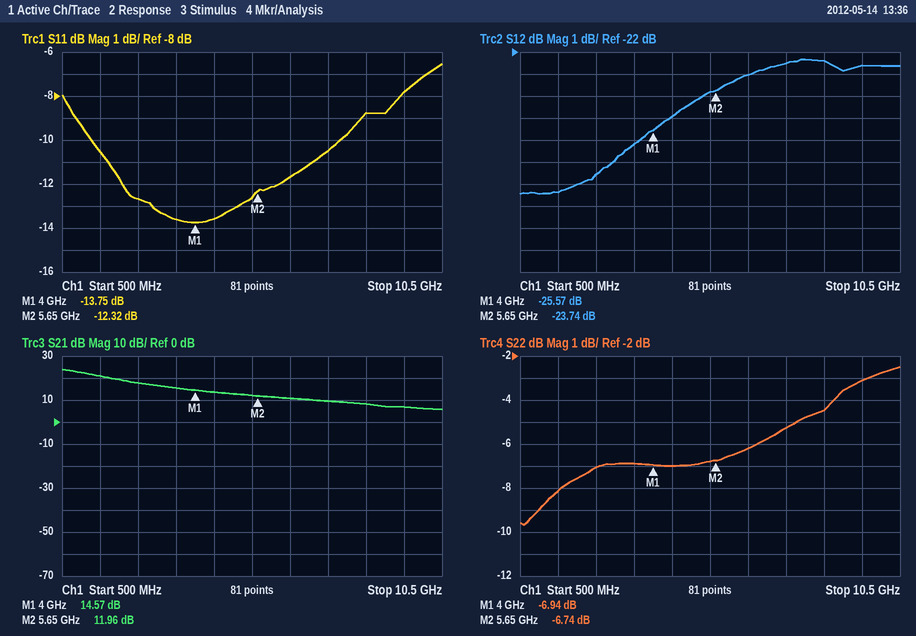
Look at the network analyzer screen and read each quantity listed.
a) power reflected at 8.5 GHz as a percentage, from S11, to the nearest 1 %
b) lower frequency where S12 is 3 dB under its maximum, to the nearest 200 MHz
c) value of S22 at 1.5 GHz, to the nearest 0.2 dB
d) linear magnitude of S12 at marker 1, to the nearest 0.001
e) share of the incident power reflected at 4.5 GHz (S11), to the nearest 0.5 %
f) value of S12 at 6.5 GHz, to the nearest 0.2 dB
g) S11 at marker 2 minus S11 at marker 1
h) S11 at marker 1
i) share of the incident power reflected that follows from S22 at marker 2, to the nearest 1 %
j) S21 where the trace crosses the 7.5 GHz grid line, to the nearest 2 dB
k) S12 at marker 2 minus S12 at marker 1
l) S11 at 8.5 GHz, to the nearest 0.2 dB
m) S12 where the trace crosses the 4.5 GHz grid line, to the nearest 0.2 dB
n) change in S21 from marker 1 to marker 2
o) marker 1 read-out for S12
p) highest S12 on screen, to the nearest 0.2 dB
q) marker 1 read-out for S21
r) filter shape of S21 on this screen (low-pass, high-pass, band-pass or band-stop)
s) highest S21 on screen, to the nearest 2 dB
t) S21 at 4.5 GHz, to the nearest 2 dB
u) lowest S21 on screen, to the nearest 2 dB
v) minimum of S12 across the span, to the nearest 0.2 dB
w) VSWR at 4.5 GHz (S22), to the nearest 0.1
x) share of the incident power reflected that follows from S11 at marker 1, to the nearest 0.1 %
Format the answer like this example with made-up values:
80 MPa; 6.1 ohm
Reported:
13 %; 4.2 GHz; -8.2 dB; 0.053; 4.5 %; -23.0 dB; 1.43 dB; -13.75 dB; 21 %; 10 dB; 1.83 dB; -8.8 dB; -25.0 dB; -2.61 dB; -25.57 dB; -22.4 dB; 14.57 dB; low-pass; 24 dB; 14 dB; 6 dB; -28.4 dB; 2.6; 4.2 %
